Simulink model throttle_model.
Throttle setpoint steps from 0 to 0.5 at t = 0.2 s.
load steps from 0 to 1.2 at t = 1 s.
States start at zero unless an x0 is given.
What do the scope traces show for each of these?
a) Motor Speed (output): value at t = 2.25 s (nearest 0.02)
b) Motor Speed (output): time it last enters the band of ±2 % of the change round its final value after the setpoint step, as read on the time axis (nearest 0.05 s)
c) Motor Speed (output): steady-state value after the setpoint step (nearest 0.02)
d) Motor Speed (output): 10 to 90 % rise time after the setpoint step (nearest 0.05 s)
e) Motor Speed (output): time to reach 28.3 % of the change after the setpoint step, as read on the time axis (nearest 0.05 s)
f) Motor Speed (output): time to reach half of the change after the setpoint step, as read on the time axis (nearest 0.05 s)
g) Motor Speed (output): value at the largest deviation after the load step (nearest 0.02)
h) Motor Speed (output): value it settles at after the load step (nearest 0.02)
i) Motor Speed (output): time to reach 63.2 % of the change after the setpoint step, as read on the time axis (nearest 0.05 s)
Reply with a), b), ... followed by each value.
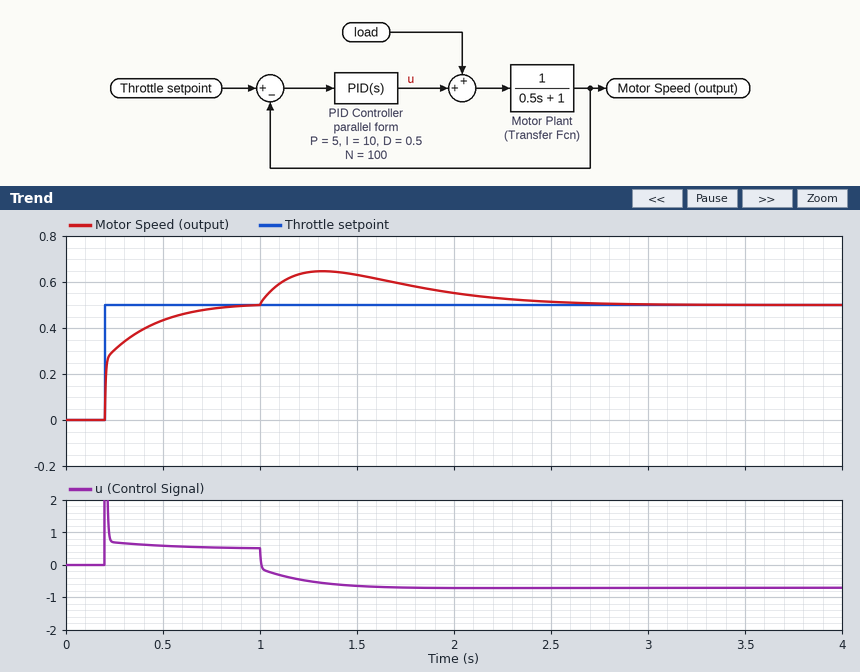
a) 0.52
b) 0.80 s
c) 0.50
d) 0.35 s
e) 0.20 s
f) 0.20 s
g) 0.64
h) 0.50
i) 0.25 s
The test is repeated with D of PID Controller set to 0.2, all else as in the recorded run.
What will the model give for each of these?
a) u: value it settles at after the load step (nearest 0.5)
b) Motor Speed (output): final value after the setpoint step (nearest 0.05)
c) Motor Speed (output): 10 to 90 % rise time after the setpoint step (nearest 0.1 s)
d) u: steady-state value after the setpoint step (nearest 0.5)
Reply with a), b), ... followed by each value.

a) -0.5
b) 0.50
c) 0.3 s
d) 0.5
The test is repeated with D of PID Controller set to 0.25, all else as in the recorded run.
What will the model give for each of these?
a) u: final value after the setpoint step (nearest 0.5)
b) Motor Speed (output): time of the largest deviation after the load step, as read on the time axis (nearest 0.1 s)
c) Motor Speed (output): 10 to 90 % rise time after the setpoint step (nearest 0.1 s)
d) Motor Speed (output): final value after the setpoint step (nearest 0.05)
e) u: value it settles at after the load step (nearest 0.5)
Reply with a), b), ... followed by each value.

a) 0.5
b) 1.3 s
c) 0.3 s
d) 0.50
e) -0.5
